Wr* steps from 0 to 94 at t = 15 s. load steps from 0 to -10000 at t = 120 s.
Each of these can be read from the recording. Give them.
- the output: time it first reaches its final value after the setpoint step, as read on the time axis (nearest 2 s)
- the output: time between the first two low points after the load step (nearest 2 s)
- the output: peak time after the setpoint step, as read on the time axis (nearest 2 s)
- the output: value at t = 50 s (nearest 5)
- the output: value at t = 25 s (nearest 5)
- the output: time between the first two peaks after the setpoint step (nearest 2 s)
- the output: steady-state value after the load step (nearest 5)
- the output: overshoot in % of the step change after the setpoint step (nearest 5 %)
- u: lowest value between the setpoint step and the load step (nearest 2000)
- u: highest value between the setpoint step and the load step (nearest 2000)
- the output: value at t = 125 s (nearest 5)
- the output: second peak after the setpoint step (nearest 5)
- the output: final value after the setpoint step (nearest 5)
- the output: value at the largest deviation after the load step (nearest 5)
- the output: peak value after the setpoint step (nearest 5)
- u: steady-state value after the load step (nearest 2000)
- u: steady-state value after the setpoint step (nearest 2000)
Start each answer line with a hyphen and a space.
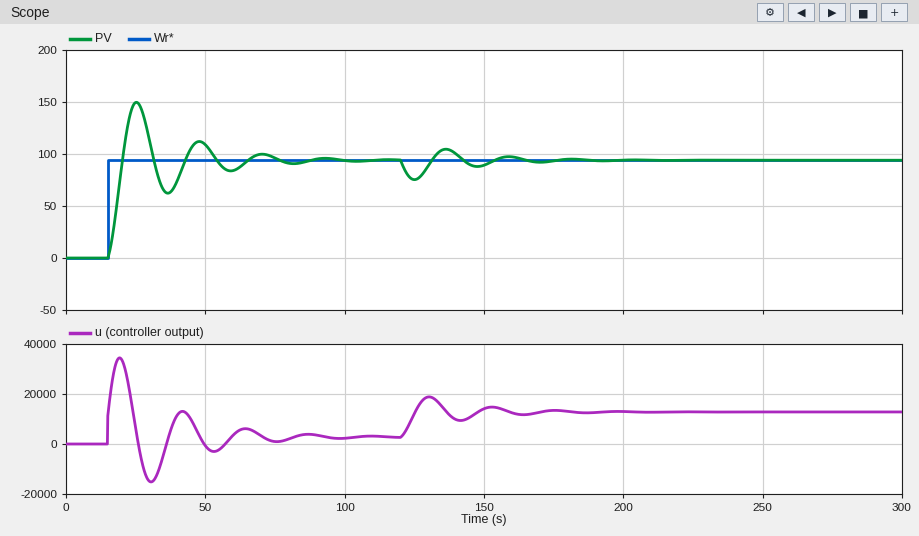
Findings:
- 20 s
- 22 s
- 26 s
- 110
- 150
- 22 s
- 95
- 60 %
- -16000
- 34000
- 75
- 110
- 95
- 75
- 150
- 12000
- 2000
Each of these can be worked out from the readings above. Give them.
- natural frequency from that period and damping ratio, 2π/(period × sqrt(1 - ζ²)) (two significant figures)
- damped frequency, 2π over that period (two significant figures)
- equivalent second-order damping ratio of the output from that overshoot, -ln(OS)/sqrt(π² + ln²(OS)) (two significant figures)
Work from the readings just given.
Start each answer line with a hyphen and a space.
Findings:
- 0.29 rad/s
- 0.29 rad/s
- 0.16
